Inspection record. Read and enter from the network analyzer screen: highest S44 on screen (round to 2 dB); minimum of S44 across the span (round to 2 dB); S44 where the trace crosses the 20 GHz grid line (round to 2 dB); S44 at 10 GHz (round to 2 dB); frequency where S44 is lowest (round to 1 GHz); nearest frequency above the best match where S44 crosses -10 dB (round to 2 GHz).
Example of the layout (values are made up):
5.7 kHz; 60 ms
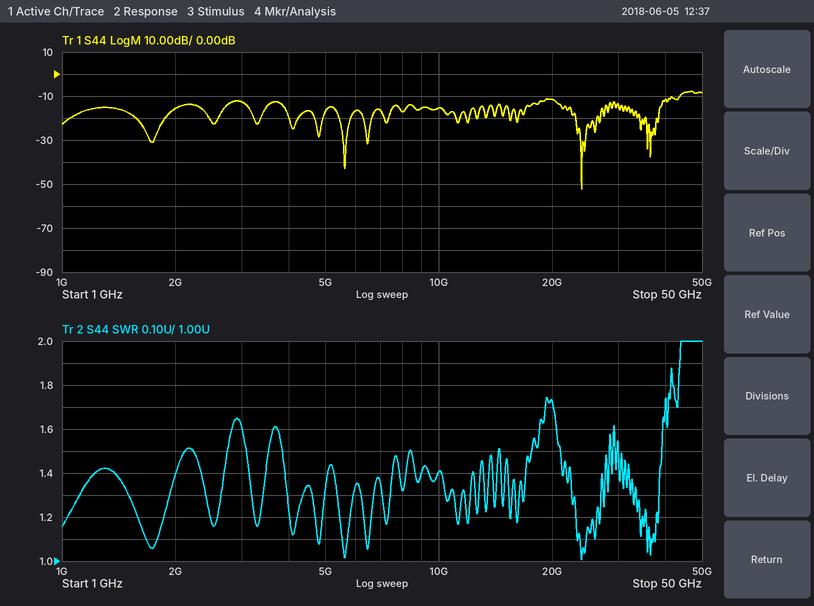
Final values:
-8 dB; -52 dB; -12 dB; -16 dB; 24 GHz; 44 GHz
